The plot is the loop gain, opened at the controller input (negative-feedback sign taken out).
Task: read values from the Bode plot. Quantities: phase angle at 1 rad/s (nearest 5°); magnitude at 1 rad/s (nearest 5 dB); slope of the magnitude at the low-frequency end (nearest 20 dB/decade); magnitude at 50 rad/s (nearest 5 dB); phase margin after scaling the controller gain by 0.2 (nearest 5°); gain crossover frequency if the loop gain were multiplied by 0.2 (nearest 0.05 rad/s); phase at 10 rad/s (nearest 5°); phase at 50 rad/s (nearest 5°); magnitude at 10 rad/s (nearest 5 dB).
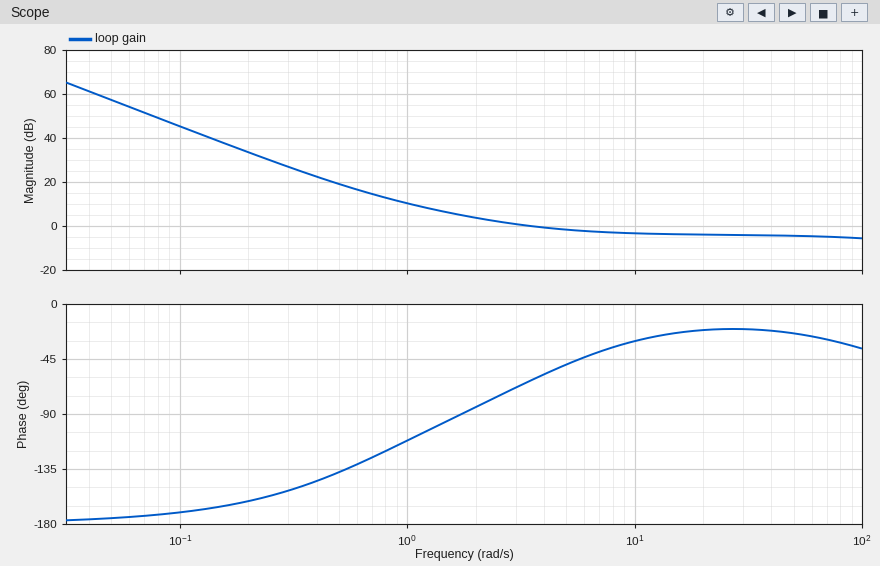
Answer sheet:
-110°
10 dB
-40 dB/decade
-5 dB
55°
0.75 rad/s
-30°
-25°
-5 dB
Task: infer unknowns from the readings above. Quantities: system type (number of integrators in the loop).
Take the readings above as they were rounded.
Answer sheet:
2
